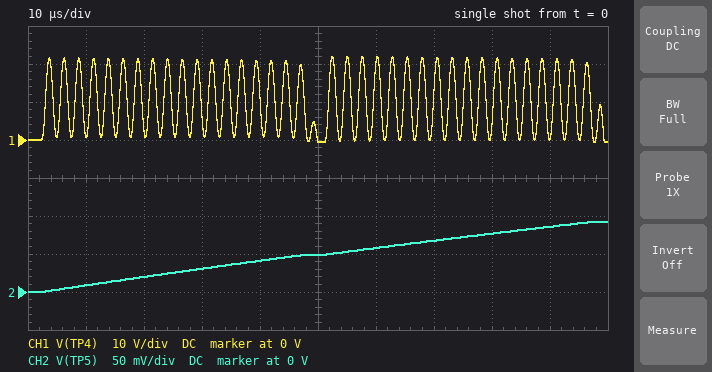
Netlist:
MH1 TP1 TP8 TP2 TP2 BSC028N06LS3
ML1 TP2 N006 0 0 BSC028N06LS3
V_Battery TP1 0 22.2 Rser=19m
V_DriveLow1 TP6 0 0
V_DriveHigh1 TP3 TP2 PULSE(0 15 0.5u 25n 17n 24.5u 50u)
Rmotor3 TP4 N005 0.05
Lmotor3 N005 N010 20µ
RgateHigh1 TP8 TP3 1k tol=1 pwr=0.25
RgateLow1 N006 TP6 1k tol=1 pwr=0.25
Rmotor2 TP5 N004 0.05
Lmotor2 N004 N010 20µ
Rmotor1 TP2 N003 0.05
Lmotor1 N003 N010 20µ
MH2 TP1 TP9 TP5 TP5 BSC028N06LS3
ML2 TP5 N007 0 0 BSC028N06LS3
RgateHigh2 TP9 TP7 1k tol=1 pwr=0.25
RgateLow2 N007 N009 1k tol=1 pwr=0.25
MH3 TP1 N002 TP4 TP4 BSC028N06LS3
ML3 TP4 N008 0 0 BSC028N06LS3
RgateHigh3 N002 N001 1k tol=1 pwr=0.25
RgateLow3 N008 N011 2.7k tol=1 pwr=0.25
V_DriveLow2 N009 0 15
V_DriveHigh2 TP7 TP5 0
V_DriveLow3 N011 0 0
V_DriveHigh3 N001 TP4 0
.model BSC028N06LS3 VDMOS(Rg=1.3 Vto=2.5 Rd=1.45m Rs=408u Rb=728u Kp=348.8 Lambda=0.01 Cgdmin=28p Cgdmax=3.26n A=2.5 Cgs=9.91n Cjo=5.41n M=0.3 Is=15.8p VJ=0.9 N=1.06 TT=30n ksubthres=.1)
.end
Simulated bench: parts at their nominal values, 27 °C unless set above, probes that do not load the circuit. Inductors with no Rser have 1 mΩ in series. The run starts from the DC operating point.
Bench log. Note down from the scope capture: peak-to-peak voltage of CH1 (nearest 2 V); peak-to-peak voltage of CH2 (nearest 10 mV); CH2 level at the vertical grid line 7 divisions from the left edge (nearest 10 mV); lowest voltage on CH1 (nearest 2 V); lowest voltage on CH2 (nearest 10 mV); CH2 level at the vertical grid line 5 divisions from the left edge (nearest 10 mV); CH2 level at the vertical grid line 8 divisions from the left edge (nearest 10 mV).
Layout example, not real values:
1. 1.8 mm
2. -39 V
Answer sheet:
1. 22 V
2. 90 mV
3. 70 mV
4. 0 V
5. 0 V
6. 50 mV
7. 80 mV
